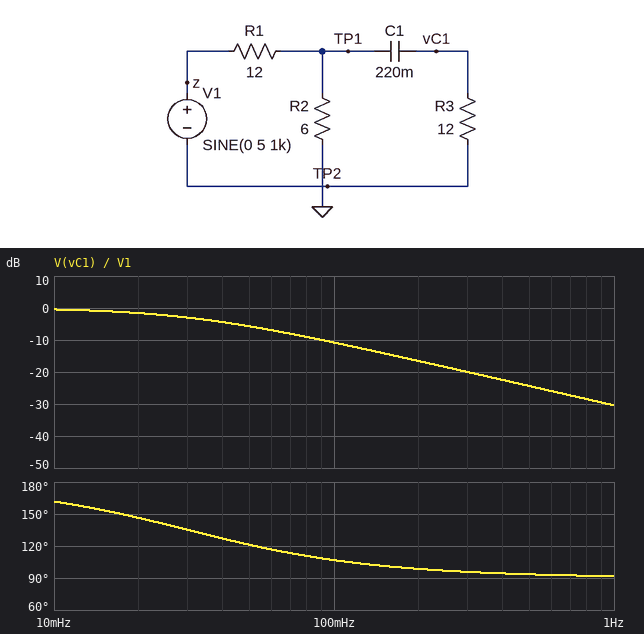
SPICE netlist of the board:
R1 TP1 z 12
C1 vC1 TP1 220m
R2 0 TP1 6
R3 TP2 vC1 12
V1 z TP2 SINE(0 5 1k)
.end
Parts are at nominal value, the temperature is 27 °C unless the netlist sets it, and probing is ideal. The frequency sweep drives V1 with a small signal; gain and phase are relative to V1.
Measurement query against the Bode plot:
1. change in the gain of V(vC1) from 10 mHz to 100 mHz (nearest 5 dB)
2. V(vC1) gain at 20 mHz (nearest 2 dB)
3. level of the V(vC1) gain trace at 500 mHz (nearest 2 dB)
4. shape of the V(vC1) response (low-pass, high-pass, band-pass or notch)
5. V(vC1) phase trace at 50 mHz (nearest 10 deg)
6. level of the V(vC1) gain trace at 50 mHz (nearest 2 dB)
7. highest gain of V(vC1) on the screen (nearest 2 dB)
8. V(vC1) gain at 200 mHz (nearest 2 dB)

-10 dB
-2 dB
-24 dB
low-pass
120 deg
-6 dB
0 dB
-16 dB
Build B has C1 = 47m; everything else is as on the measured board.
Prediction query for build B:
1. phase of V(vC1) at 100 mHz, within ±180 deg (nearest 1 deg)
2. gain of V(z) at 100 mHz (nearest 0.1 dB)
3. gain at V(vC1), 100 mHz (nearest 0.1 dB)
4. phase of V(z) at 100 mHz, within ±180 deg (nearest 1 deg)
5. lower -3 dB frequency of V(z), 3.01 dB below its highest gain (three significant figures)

145 deg
-10.8 dB
-1.8 dB
55 deg
141 mHz
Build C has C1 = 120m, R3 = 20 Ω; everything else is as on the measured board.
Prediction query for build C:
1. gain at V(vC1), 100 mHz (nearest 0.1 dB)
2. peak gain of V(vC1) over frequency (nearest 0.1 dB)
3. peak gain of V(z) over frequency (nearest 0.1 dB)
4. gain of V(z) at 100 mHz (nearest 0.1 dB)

-8.3 dB
0 dB
-8.5 dB
-9.2 dB
